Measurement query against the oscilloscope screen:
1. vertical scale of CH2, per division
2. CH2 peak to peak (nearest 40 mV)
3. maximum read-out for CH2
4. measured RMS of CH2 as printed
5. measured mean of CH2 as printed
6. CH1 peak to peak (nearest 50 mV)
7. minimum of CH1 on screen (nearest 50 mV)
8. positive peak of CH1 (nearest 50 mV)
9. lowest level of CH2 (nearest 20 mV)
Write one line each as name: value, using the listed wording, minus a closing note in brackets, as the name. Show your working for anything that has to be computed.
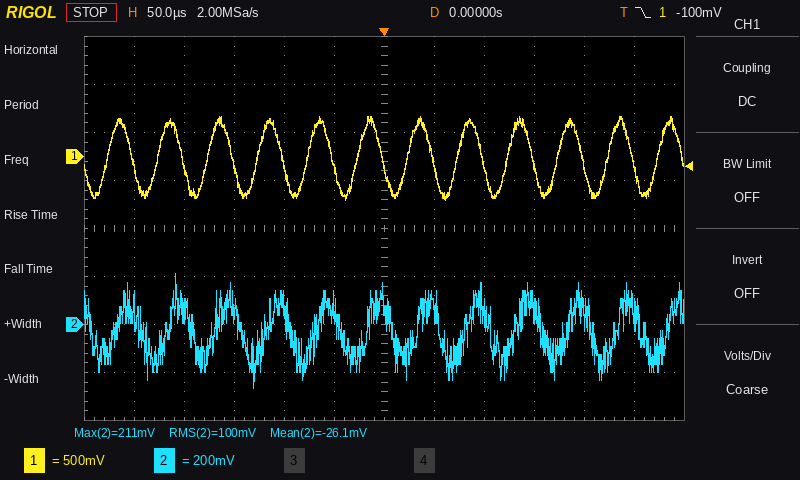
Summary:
vertical scale of CH2, per division: 200 mV
CH2 peak to peak: 480 mV
maximum read-out for CH2: 211 mV
measured RMS of CH2 as printed: 100 mV
measured mean of CH2 as printed: -26.1 mV
CH1 peak to peak: 400 mV − (-450 mV) = 850 mV
minimum of CH1 on screen: -450 mV
positive peak of CH1: 400 mV
lowest level of CH2: -260 mV
